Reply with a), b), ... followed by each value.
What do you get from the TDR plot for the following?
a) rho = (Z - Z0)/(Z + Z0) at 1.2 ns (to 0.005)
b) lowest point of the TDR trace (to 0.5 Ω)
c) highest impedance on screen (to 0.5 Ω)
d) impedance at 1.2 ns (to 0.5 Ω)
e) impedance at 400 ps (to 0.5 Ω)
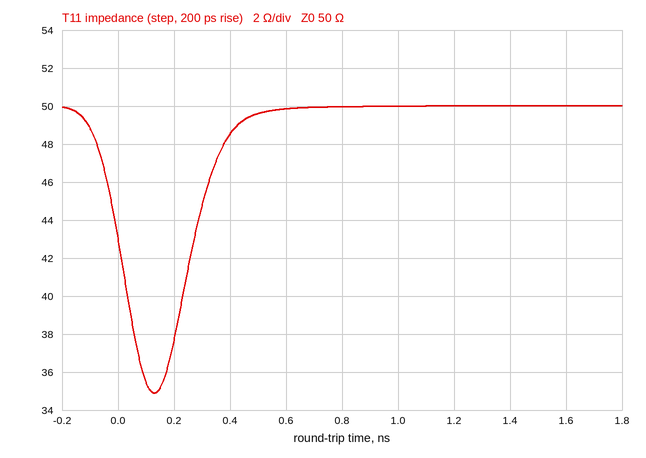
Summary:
a) 0.000
b) 35.0 Ω
c) 50.0 Ω
d) 50.0 Ω
e) 48.5 Ω
